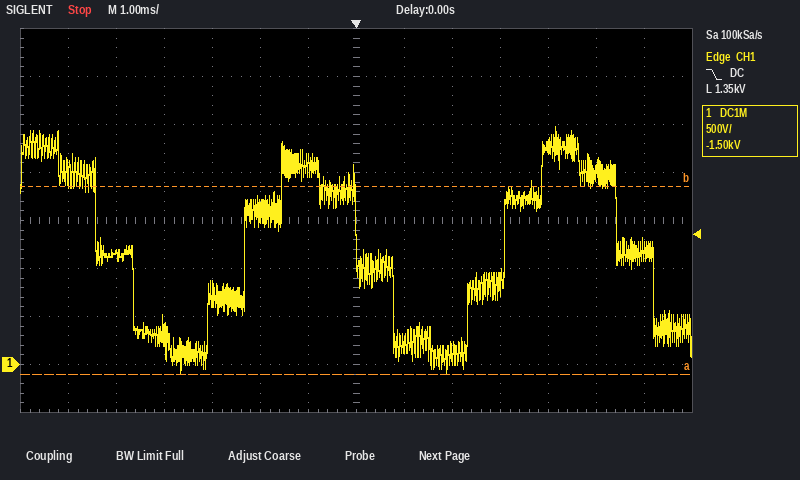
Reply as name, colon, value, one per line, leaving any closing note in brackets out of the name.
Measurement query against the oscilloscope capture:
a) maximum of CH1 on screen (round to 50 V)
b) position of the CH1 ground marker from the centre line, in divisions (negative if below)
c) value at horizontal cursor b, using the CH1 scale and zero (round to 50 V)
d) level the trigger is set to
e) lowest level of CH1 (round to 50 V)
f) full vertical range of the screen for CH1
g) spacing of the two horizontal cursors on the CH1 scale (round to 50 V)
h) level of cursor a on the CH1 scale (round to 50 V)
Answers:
maximum of CH1 on screen: 2.50 kV
position of the CH1 ground marker from the centre line, in divisions: -3.0 div
value at horizontal cursor b, using the CH1 scale and zero: 1.85 kV
level the trigger is set to: 1.35 kV
lowest level of CH1: -100 V
full vertical range of the screen for CH1: 4 kV
spacing of the two horizontal cursors on the CH1 scale: 1.95 kV
level of cursor a on the CH1 scale: -100 V
